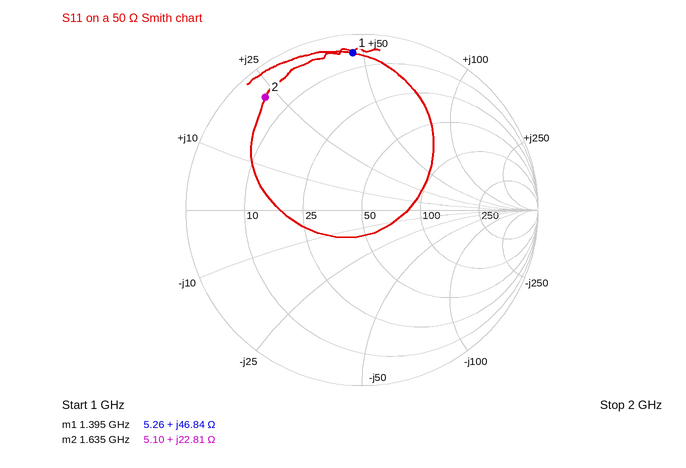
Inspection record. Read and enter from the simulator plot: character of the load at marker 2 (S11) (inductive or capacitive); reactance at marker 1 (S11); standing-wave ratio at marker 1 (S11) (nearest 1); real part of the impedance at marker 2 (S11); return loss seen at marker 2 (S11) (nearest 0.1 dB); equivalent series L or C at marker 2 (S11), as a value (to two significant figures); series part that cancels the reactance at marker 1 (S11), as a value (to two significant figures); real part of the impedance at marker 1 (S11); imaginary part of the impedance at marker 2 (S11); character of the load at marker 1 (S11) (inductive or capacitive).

inductive
+46.84 Ω
18
5.10 Ω
1.5 dB
2.2 nH
2.4 pF
5.26 Ω
+22.81 Ω
inductive
